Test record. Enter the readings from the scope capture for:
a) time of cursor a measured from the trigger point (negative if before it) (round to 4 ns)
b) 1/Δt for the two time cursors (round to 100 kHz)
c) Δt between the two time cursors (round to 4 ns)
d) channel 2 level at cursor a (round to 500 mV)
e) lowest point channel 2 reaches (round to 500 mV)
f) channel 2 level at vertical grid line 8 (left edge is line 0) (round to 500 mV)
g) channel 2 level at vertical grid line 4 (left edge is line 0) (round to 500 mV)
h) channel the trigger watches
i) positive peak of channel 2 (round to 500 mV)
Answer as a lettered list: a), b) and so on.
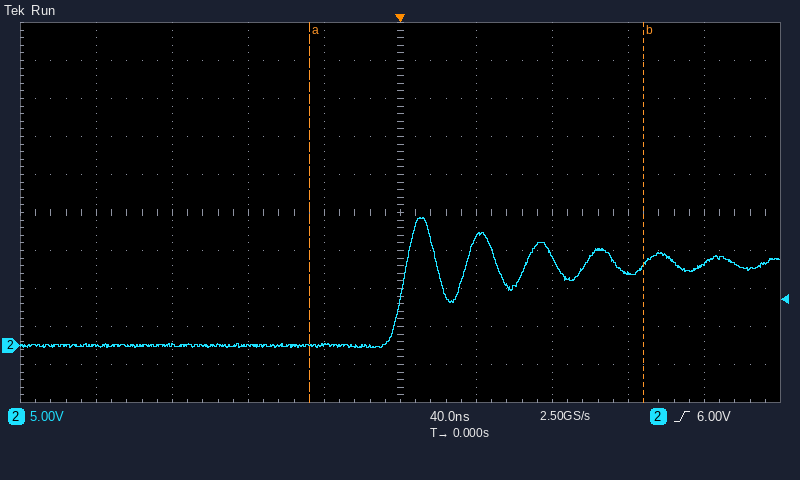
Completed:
a) -48 ns
b) 5.7 MHz
c) 176 ns
d) 0.0 V
e) -500 mV
f) 9.5 V
g) 0.0 V
h) channel 2
i) 17.0 V
